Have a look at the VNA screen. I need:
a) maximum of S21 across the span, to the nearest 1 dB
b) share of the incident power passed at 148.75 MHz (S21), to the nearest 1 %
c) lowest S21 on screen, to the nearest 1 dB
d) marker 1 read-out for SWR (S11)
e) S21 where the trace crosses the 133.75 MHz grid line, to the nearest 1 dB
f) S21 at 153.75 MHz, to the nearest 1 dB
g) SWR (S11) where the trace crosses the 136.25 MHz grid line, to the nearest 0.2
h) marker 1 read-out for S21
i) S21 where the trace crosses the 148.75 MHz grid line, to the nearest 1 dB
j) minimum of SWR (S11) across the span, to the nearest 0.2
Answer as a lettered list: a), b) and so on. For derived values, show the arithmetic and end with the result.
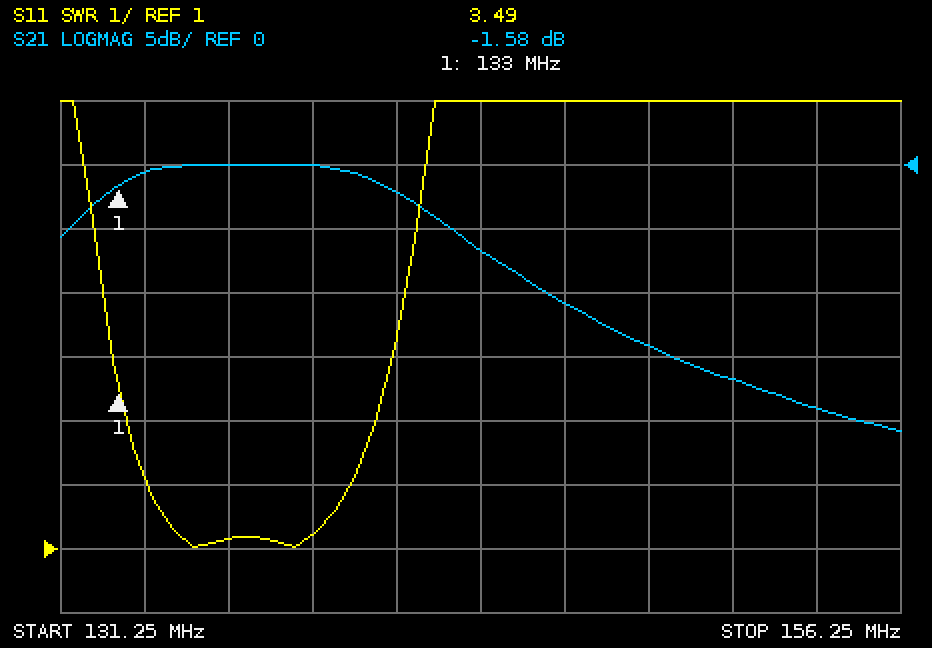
a) 0 dB
b) 10^(-14/10) ≈ 4 %
c) -21 dB
d) 3.49
e) -1 dB
f) -19 dB
g) 1.2
h) -1.58 dB
i) -14 dB
j) 1.0
